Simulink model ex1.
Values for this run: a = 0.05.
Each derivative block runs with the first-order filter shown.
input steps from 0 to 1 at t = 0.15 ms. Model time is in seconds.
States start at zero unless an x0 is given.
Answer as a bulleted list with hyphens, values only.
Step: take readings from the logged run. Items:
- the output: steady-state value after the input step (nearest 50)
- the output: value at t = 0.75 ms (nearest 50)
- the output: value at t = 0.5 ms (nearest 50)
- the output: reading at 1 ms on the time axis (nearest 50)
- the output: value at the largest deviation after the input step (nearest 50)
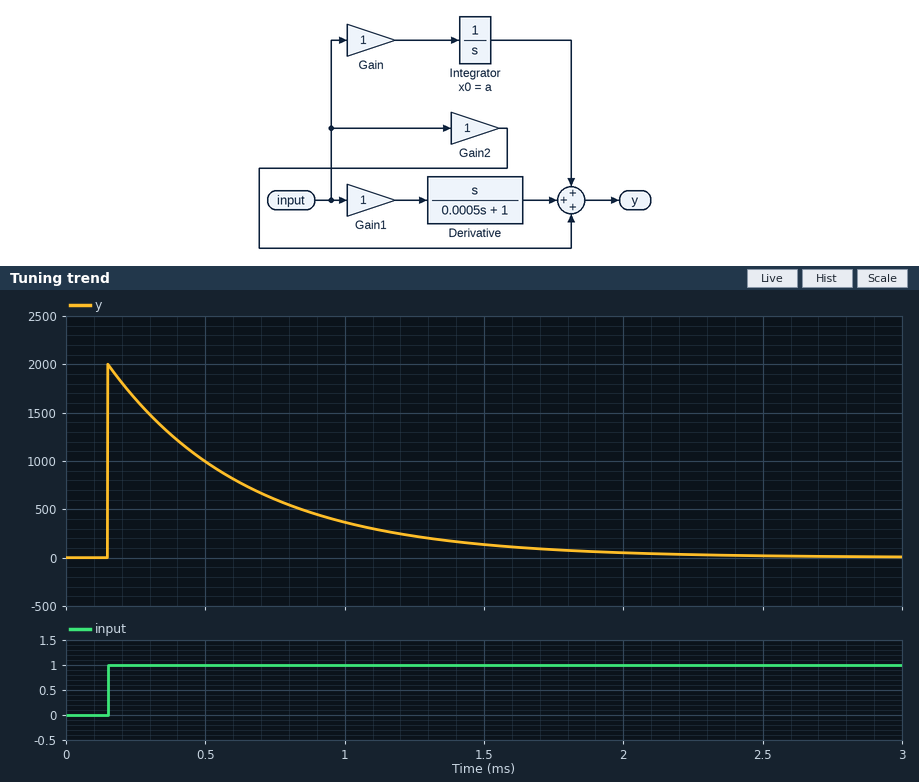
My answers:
- 0
- 600
- 1000
- 350
- 2000
